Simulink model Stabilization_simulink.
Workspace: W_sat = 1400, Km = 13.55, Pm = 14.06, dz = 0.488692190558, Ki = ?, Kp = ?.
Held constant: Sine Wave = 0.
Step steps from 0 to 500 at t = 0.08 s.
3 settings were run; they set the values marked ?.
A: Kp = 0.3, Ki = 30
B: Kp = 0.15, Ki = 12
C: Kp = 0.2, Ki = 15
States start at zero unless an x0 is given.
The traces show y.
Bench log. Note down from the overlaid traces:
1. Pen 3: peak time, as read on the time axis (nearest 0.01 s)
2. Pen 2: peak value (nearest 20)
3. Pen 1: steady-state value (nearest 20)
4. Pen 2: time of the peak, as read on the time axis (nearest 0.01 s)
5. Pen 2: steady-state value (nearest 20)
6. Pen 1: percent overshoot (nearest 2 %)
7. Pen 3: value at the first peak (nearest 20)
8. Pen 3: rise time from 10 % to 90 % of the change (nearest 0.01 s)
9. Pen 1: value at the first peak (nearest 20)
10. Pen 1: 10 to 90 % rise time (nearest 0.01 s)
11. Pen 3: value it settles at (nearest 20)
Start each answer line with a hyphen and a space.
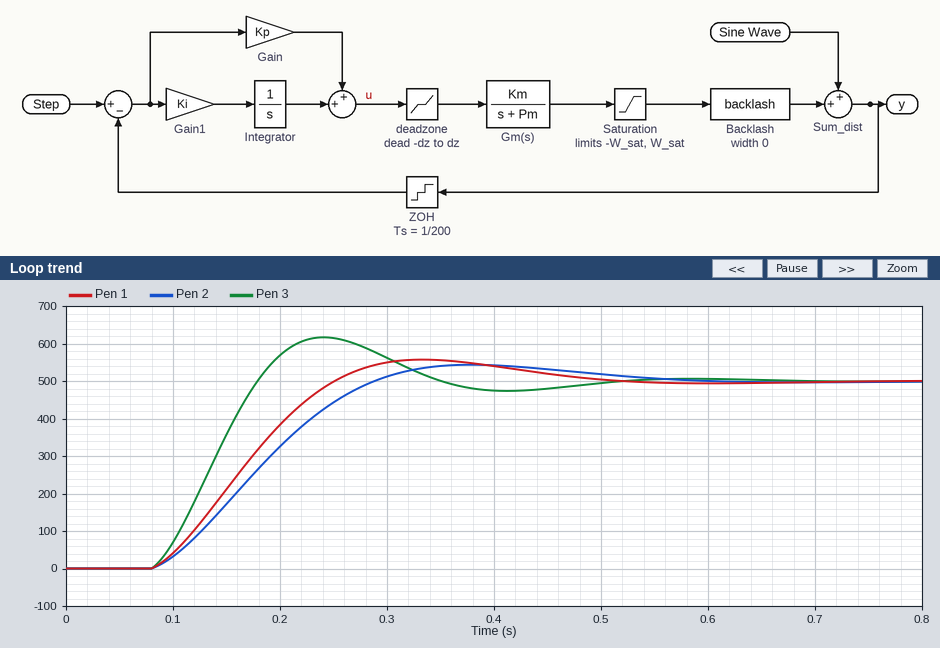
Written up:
- 0.24 s
- 540
- 500
- 0.38 s
- 500
- 12 %
- 620
- 0.07 s
- 560
- 0.12 s
- 500
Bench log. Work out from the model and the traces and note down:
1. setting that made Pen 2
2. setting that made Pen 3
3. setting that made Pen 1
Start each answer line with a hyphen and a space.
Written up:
- B
- A
- C
